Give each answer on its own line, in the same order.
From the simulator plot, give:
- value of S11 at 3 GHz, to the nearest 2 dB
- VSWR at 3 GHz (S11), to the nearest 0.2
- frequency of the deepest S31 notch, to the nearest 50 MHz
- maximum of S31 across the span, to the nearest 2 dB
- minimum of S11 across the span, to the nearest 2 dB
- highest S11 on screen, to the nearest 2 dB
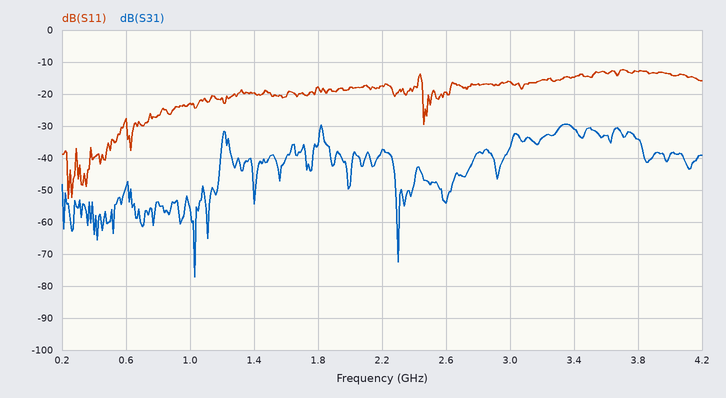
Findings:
-16 dB
1.4
1.05 GHz
-30 dB
-52 dB
-12 dB
